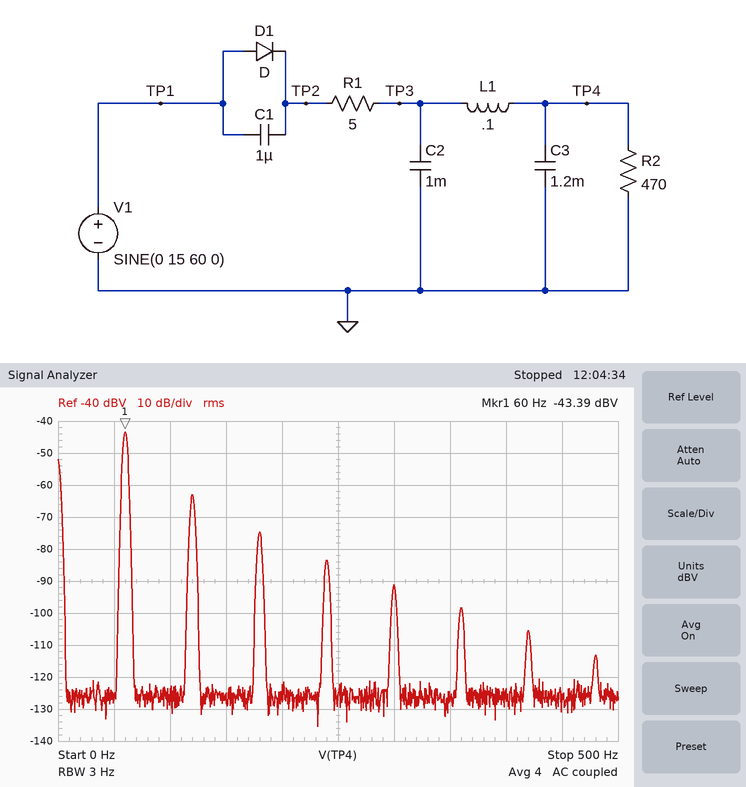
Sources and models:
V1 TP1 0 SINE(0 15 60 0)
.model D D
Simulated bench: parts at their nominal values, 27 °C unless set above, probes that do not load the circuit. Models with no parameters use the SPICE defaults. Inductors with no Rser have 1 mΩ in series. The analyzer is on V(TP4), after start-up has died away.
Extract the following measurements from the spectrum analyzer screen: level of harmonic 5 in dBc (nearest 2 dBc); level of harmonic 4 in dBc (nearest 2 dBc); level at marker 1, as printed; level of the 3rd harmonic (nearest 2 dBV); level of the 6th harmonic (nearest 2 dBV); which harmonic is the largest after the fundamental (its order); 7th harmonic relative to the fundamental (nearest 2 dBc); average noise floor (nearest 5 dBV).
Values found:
-48 dBc
-40 dBc
-43.39 dBV
-74 dBV
-98 dBV
2
-62 dBc
-125 dBV
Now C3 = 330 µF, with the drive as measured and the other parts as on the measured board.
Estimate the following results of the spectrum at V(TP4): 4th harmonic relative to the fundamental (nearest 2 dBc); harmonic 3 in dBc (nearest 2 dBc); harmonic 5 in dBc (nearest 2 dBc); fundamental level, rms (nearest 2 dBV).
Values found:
-42 dBc
-32 dBc
-50 dBc
-30 dBV
